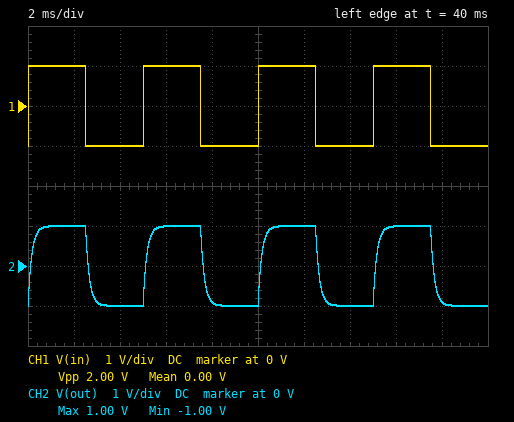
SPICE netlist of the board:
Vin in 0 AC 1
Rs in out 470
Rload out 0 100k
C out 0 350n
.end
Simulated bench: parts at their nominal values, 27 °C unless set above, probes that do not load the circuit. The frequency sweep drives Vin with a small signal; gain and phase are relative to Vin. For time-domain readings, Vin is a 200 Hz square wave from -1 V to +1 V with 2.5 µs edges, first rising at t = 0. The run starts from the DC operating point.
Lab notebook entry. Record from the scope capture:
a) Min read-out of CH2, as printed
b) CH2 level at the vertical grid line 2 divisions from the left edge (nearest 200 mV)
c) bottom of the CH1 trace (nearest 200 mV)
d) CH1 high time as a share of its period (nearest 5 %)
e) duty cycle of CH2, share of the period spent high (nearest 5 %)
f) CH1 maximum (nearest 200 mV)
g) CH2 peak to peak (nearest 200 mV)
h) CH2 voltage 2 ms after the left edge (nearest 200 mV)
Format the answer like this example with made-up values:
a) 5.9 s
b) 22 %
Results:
a) -1.00 V
b) -1.0 V
c) -1.0 V
d) 50 %
e) 50 %
f) 1.0 V
g) 2.0 V
h) 1.0 V
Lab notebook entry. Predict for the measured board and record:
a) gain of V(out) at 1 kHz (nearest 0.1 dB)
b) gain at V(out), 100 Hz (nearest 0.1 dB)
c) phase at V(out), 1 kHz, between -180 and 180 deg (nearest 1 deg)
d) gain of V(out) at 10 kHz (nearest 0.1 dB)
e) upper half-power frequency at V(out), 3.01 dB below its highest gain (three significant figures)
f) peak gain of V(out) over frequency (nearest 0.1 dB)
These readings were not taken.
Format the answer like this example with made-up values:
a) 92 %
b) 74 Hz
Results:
a) -3.2 dB
b) -0.1 dB
c) -46 deg
d) -20.3 dB
e) 972 Hz
f) 0 dB
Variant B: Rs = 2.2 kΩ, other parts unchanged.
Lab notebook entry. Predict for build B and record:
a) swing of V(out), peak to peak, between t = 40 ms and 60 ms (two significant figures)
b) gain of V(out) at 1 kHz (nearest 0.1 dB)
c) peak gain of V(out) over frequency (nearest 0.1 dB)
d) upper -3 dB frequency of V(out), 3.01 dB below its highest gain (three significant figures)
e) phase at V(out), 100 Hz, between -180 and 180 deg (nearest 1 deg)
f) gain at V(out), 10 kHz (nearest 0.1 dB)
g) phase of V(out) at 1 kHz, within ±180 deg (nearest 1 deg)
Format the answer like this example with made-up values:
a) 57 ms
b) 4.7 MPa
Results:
a) 1.8 V
b) -13.9 dB
c) -0.2 dB
d) 211 Hz
e) -25 deg
f) -33.7 dB
g) -78 deg
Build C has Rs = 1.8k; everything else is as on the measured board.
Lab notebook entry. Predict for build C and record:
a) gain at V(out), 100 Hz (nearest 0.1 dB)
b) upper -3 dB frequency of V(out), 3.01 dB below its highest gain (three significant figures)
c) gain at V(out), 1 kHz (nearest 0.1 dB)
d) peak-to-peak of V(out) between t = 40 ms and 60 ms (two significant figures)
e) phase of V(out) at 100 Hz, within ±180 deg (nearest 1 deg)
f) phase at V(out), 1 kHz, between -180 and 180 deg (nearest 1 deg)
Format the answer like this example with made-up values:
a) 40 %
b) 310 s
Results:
a) -0.8 dB
b) 257 Hz
c) -12.2 dB
d) 1.9 V
e) -21 deg
f) -76 deg
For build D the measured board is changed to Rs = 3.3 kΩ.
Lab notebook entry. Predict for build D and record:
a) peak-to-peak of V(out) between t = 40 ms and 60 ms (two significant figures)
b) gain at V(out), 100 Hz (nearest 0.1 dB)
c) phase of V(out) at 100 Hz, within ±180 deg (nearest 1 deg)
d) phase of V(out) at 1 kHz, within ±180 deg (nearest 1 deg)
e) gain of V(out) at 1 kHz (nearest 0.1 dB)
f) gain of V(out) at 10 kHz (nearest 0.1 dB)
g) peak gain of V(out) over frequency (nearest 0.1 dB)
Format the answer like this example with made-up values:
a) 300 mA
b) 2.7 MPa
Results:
a) 1.6 V
b) -2.0 dB
c) -35 deg
d) -82 deg
e) -17.3 dB
f) -37.2 dB
g) -0.3 dB
